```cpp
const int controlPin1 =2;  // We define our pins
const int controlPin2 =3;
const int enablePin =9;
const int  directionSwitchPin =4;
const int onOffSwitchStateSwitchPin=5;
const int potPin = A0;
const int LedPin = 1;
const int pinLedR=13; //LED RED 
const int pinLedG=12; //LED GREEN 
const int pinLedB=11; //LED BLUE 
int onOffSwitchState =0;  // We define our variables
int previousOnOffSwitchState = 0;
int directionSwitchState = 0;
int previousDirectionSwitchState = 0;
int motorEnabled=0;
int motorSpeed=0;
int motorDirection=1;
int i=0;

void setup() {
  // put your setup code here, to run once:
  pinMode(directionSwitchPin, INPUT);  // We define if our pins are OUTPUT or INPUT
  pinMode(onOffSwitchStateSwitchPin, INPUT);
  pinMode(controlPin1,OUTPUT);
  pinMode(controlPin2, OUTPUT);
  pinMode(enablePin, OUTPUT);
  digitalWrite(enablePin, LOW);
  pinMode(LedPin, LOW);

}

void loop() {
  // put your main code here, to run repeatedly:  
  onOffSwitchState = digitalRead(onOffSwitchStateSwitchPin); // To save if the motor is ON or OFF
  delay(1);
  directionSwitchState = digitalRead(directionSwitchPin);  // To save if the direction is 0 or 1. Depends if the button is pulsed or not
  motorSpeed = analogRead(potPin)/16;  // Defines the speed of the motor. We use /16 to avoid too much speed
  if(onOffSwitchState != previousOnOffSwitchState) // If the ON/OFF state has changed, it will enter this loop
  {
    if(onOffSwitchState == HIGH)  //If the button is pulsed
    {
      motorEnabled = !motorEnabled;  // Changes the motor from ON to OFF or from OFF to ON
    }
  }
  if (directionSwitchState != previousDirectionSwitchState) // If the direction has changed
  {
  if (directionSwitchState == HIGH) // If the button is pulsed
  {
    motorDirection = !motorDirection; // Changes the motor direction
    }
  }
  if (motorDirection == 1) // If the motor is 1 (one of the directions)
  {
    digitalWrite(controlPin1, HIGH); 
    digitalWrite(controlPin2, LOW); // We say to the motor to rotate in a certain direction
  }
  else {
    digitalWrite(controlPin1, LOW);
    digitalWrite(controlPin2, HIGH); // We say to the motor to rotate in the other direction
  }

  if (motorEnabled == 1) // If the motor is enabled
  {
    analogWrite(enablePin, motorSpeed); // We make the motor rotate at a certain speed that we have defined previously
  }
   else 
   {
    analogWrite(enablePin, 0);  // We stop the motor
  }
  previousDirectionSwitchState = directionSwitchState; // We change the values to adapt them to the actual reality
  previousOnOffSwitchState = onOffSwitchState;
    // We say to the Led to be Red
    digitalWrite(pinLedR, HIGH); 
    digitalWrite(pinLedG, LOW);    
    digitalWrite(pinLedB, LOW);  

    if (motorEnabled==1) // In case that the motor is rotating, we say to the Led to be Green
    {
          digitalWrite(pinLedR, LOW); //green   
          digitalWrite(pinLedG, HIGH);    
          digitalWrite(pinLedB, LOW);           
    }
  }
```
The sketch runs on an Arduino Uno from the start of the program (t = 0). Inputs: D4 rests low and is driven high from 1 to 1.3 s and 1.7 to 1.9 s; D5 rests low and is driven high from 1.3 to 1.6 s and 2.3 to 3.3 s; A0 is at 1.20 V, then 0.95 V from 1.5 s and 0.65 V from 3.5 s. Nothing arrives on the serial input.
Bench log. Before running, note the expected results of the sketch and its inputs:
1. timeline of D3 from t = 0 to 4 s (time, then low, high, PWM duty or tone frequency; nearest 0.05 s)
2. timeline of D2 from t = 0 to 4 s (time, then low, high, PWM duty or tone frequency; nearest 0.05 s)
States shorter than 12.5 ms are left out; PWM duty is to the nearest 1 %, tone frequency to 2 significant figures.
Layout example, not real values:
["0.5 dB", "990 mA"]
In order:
["0 s low; 1 s high; 1.7 s low", "0 s high; 1 s low; 1.7 s high"]
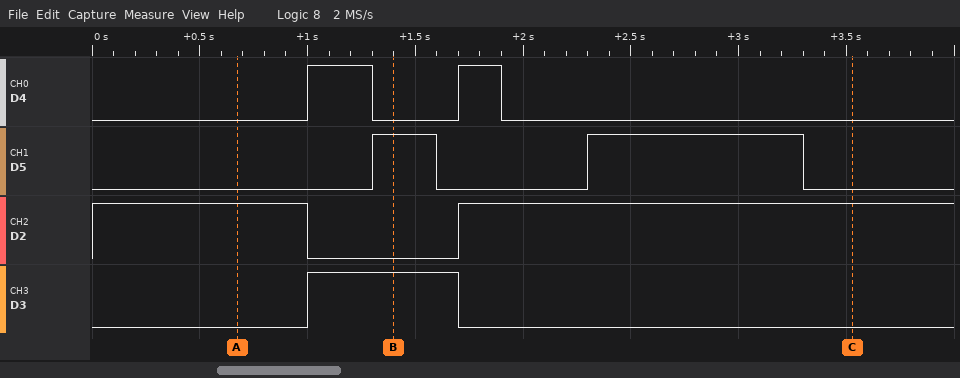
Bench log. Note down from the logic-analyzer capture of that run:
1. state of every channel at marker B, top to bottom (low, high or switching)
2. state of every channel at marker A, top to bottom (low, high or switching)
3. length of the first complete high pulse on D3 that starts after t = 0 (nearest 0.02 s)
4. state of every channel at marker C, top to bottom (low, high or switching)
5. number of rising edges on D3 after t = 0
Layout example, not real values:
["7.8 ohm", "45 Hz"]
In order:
["D4 low, D5 high, D2 low, D3 high", "D4 low, D5 low, D2 high, D3 low", "0.70 s", "D4 low, D5 low, D2 high, D3 low", "1"]
